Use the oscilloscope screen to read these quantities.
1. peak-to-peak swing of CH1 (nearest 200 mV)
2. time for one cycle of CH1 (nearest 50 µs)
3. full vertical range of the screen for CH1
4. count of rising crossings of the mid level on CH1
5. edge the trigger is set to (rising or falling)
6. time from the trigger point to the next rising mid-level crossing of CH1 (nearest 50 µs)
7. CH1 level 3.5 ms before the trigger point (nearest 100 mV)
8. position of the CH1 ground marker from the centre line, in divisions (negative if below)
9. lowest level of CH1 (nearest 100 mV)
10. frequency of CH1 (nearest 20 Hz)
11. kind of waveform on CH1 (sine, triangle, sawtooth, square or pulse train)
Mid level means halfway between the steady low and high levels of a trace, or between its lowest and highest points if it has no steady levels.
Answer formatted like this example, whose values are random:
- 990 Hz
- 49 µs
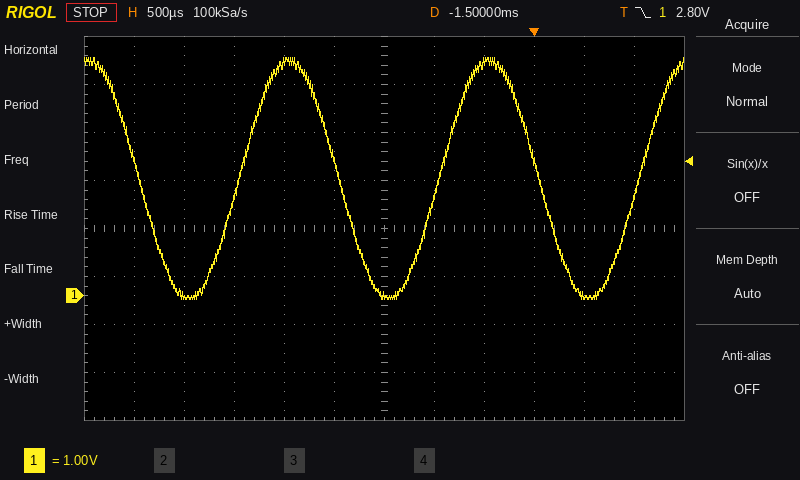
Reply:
- 5.0 V
- 2.00 ms
- 8 V
- 3
- falling
- 1.05 ms
- 0.0 V
- -1.4 div
- -100 mV
- 500 Hz
- sine
